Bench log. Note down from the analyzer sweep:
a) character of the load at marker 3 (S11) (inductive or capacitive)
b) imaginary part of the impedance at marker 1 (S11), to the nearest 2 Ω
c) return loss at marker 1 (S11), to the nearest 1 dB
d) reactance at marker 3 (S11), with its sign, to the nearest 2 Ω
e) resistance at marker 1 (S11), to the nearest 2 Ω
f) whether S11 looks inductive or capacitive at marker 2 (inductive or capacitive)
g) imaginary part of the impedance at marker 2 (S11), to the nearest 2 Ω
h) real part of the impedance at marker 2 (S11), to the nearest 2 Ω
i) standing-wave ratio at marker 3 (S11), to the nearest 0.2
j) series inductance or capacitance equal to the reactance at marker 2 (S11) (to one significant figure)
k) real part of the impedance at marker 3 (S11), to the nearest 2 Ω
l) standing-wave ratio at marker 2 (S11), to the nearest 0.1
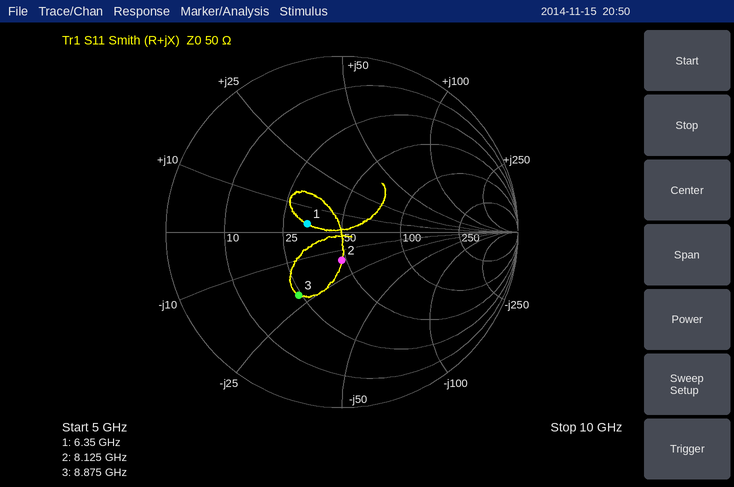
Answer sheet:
capacitive
+4 Ω
14 dB
-22 Ω
34 Ω
capacitive
-16 Ω
48 Ω
2.6
1 pF
24 Ω
1.4
